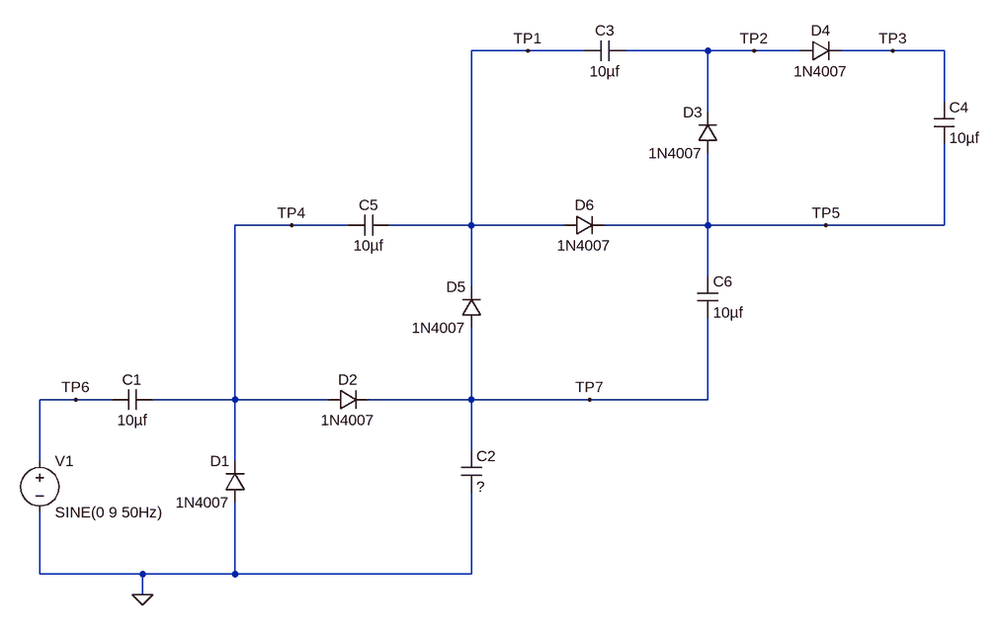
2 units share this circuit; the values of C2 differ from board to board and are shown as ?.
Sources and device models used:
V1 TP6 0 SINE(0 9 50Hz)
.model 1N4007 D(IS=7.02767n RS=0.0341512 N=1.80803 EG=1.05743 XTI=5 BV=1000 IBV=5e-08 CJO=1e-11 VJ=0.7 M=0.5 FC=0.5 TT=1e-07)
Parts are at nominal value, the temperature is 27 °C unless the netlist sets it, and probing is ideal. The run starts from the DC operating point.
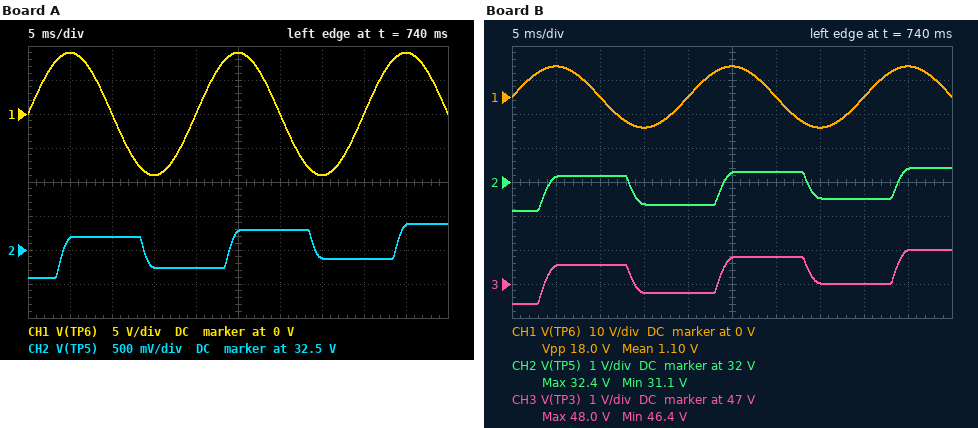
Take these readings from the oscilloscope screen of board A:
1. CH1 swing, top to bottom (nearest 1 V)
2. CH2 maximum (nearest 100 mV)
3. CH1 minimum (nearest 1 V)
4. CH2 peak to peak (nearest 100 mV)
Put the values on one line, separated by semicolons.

18 V; 32.9 V; -9 V; 800 mV
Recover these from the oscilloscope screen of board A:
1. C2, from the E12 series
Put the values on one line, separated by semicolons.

12 µF
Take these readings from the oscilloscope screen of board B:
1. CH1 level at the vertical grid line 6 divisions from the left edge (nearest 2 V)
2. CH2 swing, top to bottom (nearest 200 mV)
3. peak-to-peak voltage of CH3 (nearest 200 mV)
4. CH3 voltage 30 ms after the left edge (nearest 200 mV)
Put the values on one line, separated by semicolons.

0 V; 1.2 V; 1.6 V; 47.8 V
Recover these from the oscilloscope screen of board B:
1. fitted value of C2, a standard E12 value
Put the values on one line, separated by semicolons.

6.8 µF
